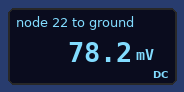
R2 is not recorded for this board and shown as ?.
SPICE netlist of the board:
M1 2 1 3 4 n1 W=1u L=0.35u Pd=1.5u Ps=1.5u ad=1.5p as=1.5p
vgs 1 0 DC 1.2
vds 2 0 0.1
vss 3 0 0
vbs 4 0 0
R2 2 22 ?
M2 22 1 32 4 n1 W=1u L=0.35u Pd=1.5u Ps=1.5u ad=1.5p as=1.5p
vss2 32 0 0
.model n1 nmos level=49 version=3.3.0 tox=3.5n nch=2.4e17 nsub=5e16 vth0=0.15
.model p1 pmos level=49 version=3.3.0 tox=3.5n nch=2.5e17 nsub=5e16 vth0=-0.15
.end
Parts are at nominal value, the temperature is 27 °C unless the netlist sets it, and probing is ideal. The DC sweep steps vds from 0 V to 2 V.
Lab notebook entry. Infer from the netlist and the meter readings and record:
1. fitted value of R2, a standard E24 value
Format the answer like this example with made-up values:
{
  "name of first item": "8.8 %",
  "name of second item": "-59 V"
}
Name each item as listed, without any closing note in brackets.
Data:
{
  "fitted value of R2, a standard E24 value": "430 Ω"
}
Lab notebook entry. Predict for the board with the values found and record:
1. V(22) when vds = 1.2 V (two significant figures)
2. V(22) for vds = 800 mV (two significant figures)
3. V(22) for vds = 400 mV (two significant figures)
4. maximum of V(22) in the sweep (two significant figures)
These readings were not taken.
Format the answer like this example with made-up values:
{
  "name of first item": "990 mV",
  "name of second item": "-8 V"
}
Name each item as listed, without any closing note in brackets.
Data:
{
  "V(22) when vds = 1.2 V": "1.1 V",
  "V(22) for vds = 800 mV": "720 mV",
  "V(22) for vds = 400 mV": "330 mV",
  "maximum of V(22) in the sweep": "1.9 V"
}
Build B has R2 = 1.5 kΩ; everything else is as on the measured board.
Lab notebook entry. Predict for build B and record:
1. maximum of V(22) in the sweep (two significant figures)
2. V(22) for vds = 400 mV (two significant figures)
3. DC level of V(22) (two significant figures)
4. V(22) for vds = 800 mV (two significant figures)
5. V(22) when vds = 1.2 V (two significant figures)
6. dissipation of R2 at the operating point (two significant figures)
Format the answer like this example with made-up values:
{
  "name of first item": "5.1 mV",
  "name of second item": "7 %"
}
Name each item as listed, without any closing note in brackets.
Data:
{
  "maximum of V(22) in the sweep": "1.7 V",
  "V(22) for vds = 400 mV": "220 mV",
  "DC level of V(22)": "50 mV",
  "V(22) for vds = 800 mV": "530 mV",
  "V(22) when vds = 1.2 V": "910 mV",
  "dissipation of R2 at the operating point": "1.7 µW"
}
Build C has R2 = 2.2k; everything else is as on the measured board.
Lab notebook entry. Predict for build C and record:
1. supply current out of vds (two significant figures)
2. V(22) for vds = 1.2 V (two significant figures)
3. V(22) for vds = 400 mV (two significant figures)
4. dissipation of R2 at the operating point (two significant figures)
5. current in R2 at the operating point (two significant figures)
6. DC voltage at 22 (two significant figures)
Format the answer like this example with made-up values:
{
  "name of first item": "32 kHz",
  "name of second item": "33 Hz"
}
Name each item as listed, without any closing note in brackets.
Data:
{
  "supply current out of vds": "90 µA",
  "V(22) for vds = 1.2 V": "780 mV",
  "V(22) for vds = 400 mV": "180 mV",
  "dissipation of R2 at the operating point": "1.6 µW",
  "current in R2 at the operating point": "27 µA",
  "DC voltage at 22": "40 mV"
}
